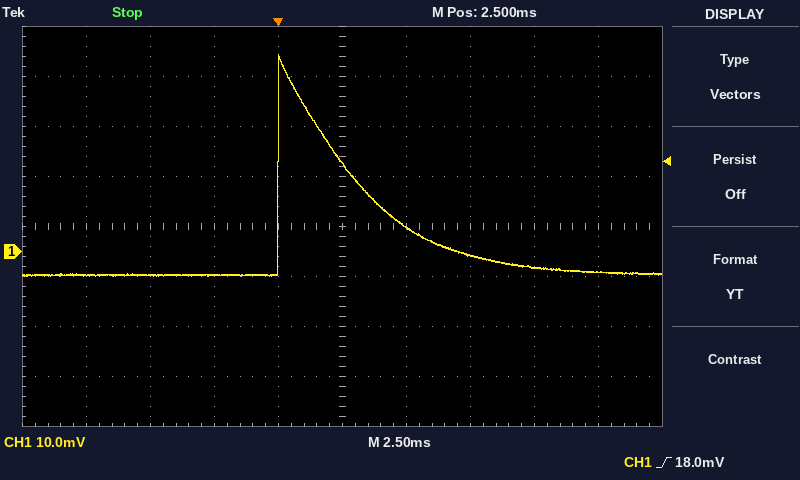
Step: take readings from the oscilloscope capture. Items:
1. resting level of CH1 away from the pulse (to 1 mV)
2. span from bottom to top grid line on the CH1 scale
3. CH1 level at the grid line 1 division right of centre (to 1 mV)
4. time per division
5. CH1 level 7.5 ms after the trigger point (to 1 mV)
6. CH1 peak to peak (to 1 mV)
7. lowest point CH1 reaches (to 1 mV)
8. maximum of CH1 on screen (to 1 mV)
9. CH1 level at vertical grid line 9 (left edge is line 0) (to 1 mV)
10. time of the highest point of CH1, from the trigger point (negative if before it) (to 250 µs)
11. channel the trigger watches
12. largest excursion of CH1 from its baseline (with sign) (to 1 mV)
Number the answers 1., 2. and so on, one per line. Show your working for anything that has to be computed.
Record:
1. -5 mV
2. 80 mV
3. 5 mV
4. 2.5 ms
5. -1 mV
6. 39 mV − (-5 mV) = 44 mV
7. -5 mV
8. 39 mV
9. -4 mV
10. 0.00 ms
11. CH1
12. 39 mV − (-5 mV) = +44 mV
